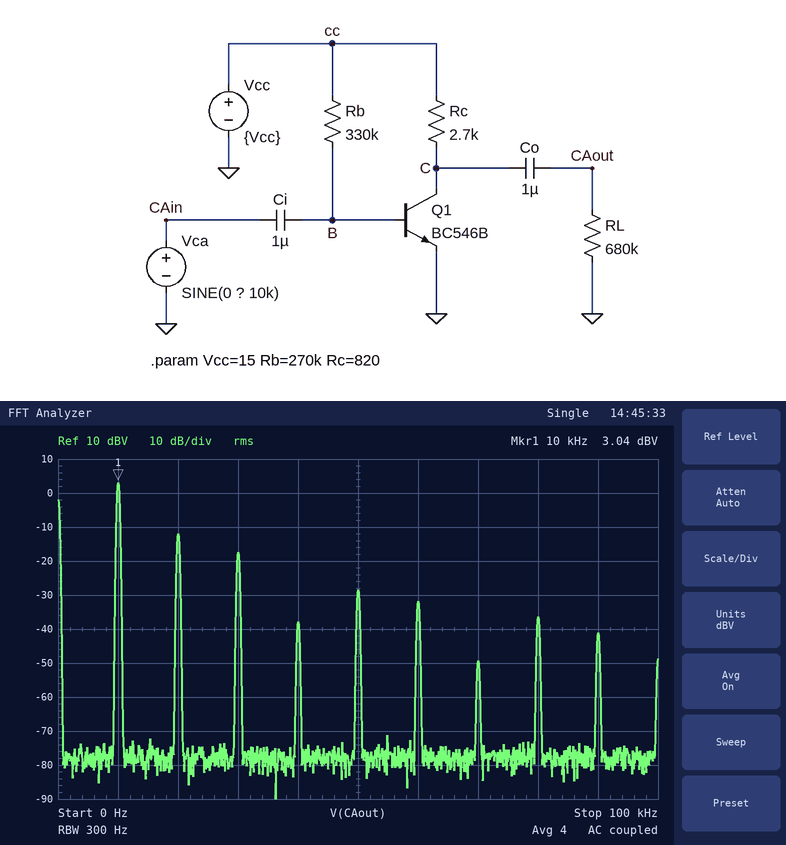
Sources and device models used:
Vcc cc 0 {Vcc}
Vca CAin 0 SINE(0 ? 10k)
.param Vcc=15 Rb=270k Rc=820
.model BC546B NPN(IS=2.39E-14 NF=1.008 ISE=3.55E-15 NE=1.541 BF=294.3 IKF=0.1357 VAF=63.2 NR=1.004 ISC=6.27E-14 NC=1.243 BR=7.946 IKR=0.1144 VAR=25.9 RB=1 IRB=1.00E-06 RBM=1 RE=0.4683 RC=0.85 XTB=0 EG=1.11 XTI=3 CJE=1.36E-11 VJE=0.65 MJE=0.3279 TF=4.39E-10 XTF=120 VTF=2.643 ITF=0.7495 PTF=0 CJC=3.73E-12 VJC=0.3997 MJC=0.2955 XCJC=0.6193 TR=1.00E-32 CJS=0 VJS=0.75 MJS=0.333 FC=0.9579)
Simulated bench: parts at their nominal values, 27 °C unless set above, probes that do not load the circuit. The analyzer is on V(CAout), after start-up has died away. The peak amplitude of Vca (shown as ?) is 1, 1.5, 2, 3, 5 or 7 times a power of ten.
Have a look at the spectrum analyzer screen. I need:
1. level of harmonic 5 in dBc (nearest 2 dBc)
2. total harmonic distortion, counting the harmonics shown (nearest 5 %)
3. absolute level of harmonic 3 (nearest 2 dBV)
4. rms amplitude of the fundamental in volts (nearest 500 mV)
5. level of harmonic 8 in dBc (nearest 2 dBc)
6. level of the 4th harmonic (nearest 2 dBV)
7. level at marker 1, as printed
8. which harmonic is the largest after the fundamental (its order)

-32 dBc
20 %
-18 dBV
1.5 V
-40 dBc
-38 dBV
3.04 dBV
2
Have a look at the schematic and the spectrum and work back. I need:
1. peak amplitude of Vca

7 mV
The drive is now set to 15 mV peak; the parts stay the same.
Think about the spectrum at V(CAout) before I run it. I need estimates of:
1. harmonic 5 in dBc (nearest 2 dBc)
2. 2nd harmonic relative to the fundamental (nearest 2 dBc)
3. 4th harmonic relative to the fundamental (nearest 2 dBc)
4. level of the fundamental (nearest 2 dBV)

-44 dBc
-26 dBc
-28 dBc
10 dBV
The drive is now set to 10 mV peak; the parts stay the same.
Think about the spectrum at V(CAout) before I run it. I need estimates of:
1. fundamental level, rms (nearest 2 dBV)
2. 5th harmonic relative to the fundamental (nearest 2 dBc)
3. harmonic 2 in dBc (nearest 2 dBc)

6 dBV
-38 dBc
-18 dBc
